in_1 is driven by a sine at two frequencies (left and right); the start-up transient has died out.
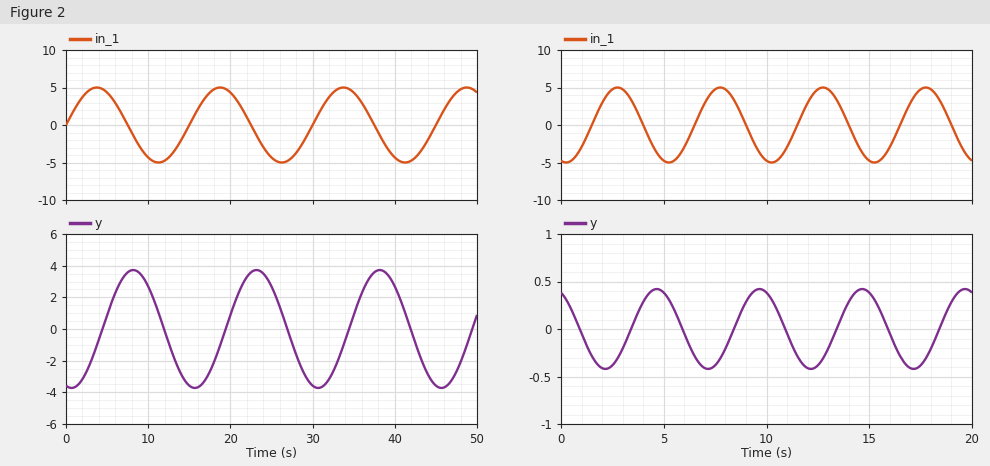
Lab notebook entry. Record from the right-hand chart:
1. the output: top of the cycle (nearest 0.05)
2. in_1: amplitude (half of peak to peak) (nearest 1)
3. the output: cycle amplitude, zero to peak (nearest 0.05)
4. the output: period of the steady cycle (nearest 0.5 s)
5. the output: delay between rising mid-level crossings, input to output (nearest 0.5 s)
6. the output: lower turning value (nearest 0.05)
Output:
0.40
5
0.40
5.0 s
2.0 s
-0.40
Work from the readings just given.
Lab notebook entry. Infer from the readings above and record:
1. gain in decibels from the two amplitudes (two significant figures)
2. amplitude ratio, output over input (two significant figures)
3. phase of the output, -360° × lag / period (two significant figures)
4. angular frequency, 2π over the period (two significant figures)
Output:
-22 dB
0.080
-140°
1.3 rad/s
